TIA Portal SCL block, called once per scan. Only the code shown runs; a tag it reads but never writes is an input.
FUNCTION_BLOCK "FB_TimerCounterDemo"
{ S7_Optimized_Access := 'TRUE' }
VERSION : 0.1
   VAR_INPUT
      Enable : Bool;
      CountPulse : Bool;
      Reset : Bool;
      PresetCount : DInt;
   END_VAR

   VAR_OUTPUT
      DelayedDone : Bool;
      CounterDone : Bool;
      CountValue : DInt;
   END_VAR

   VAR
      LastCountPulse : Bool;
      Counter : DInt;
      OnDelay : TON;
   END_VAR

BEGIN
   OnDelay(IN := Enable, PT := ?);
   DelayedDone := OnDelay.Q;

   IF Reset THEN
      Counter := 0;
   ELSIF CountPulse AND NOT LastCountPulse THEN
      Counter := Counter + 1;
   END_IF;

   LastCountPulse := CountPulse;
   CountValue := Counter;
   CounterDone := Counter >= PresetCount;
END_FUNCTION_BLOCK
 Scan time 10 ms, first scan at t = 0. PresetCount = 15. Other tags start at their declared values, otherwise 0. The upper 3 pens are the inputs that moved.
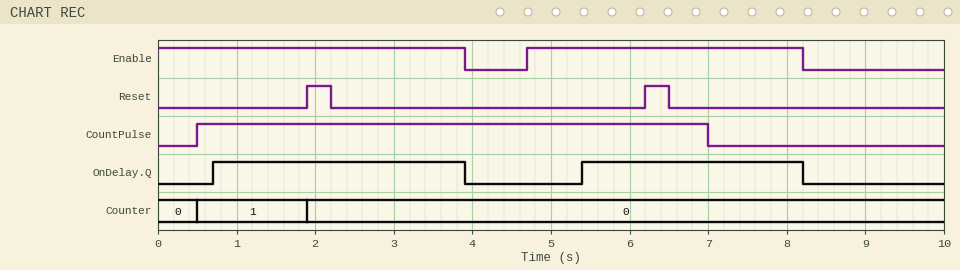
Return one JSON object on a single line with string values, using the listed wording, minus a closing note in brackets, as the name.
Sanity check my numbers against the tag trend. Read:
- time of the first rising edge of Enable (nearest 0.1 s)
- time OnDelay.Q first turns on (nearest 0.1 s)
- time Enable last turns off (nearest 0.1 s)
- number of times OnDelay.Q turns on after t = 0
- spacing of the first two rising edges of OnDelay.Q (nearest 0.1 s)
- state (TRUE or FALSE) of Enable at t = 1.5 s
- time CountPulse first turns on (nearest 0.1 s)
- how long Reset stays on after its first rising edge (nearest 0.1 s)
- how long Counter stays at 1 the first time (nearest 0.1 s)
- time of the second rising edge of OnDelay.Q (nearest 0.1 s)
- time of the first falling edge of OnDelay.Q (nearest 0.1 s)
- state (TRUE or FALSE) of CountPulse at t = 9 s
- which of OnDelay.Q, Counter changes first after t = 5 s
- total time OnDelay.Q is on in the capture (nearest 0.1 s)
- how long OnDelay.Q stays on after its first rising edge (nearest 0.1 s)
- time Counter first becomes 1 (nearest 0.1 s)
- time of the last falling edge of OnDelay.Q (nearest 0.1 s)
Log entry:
{"time of the first rising edge of Enable": "4.7 s", "time OnDelay.Q first turns on": "0.7 s", "time Enable last turns off": "8.2 s", "number of times OnDelay.Q turns on after t = 0": "2", "spacing of the first two rising edges of OnDelay.Q": "4.7 s", "state (TRUE or FALSE) of Enable at t = 1.5 s": "TRUE", "time CountPulse first turns on": "0.5 s", "how long Reset stays on after its first rising edge": "0.3 s", "how long Counter stays at 1 the first time": "1.4 s", "time of the second rising edge of OnDelay.Q": "5.4 s", "time of the first falling edge of OnDelay.Q": "3.9 s", "state (TRUE or FALSE) of CountPulse at t = 9 s": "FALSE", "which of OnDelay.Q, Counter changes first after t = 5 s": "OnDelay.Q", "total time OnDelay.Q is on in the capture": "6.0 s", "how long OnDelay.Q stays on after its first rising edge": "3.2 s", "time Counter first becomes 1": "0.5 s", "time of the last falling edge of OnDelay.Q": "8.2 s"}
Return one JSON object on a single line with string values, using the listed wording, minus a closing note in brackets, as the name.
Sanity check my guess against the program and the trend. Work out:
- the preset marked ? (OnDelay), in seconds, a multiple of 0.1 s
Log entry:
{"the preset marked ? (OnDelay), in seconds, a multiple of 0.1 s": "0.7 s"}
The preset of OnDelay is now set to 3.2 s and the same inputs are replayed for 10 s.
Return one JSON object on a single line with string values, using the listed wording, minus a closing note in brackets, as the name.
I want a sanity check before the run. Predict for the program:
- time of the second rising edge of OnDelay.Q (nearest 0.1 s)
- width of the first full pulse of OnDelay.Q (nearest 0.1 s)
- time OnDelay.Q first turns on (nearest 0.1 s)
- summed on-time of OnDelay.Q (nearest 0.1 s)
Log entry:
{"time of the second rising edge of OnDelay.Q": "7.9 s", "width of the first full pulse of OnDelay.Q": "0.7 s", "time OnDelay.Q first turns on": "3.2 s", "summed on-time of OnDelay.Q": "1.0 s"}
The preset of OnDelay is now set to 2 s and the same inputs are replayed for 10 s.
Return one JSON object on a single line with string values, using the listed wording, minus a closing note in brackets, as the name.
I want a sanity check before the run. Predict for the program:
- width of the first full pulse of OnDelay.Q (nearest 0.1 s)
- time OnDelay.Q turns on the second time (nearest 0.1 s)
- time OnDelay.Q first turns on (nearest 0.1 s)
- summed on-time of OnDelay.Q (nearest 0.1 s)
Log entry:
{"width of the first full pulse of OnDelay.Q": "1.9 s", "time OnDelay.Q turns on the second time": "6.7 s", "time OnDelay.Q first turns on": "2.0 s", "summed on-time of OnDelay.Q": "3.4 s"}
